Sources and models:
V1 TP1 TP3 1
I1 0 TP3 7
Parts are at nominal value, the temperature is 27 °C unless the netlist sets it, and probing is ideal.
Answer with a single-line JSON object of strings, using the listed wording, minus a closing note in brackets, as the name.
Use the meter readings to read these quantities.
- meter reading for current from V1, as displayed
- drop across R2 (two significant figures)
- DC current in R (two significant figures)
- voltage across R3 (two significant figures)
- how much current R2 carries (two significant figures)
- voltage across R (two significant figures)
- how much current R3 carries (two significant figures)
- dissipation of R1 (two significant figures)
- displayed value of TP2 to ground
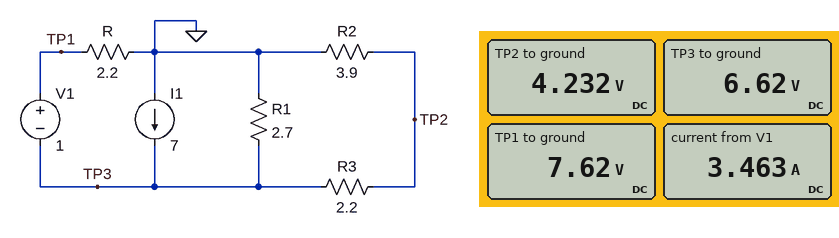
{"meter reading for current from V1, as displayed": "3.463 A", "drop across R2": "4.2 V", "DC current in R": "3.5 A", "voltage across R3": "2.4 V", "how much current R2 carries": "1.1 A", "voltage across R": "7.6 V", "how much current R3 carries": "1.1 A", "dissipation of R1": "16 W", "displayed value of TP2 to ground": "4.232 V"}
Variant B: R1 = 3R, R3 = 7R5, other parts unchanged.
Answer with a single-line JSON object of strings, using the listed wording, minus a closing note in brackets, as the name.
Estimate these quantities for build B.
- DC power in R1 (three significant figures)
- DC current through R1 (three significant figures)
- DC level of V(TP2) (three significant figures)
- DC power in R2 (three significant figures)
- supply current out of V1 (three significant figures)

{"DC power in R1": "18.6 W", "DC current through R1": "2.49 A", "DC level of V(TP2)": "2.56 V", "DC power in R2": "1.68 W", "supply current out of V1": "3.85 A"}
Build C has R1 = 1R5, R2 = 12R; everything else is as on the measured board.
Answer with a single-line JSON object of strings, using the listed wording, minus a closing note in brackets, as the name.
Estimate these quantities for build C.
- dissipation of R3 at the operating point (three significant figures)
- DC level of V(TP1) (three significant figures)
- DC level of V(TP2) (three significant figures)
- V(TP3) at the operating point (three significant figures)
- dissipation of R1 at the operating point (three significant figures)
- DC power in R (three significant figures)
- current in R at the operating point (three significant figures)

{"dissipation of R3 at the operating point": "329 mW", "DC level of V(TP1)": "6.49 V", "DC level of V(TP2)": "4.64 V", "V(TP3) at the operating point": "5.49 V", "dissipation of R1 at the operating point": "20.1 W", "DC power in R": "19.2 W", "current in R at the operating point": "2.95 A"}
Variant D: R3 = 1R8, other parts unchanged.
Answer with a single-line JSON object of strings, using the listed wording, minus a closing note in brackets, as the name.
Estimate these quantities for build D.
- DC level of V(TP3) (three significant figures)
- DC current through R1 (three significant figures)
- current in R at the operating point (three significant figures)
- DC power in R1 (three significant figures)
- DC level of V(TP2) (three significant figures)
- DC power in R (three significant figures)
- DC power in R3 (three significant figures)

{"DC level of V(TP3)": "6.54 V", "DC current through R1": "2.42 A", "current in R at the operating point": "3.43 A", "DC power in R1": "15.9 W", "DC level of V(TP2)": "4.48 V", "DC power in R": "25.9 W", "DC power in R3": "2.37 W"}
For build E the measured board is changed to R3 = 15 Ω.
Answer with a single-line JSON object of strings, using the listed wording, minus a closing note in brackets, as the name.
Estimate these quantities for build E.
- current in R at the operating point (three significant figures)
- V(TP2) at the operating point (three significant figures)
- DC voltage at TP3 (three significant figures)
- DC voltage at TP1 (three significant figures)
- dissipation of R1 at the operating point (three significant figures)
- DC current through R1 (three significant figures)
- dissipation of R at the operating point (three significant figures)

{"current in R at the operating point": "3.84 A", "V(TP2) at the operating point": "1.54 V", "DC voltage at TP3": "7.46 V", "DC voltage at TP1": "8.46 V", "dissipation of R1 at the operating point": "20.6 W", "DC current through R1": "2.76 A", "dissipation of R at the operating point": "32.5 W"}
